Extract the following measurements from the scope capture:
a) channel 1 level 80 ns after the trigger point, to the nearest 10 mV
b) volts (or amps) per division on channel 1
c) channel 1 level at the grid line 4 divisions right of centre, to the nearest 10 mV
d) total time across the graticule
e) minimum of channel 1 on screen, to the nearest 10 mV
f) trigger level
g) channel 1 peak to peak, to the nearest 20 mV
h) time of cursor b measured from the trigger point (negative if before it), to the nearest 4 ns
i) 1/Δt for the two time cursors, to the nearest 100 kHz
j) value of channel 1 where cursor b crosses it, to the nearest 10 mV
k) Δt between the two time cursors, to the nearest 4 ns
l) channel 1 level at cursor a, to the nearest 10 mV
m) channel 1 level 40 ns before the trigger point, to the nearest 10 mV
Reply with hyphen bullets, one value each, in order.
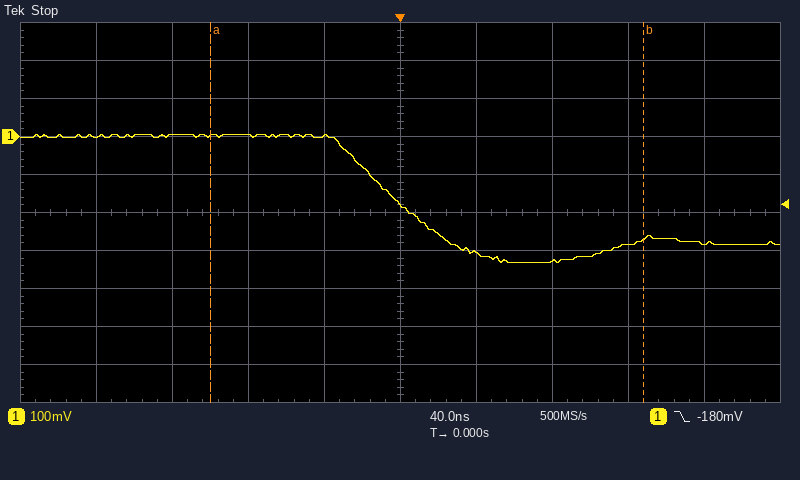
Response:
- -330 mV
- 100 mV
- -280 mV
- 400 ns
- -330 mV
- -180 mV
- 340 mV
- +128 ns
- 4.4 MHz
- -270 mV
- 228 ns
- 0 mV
- 0 mV
